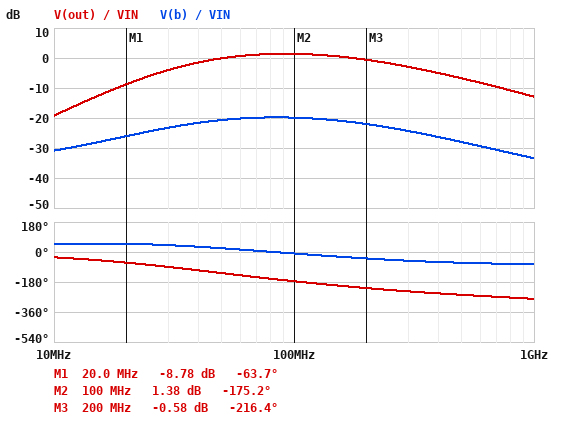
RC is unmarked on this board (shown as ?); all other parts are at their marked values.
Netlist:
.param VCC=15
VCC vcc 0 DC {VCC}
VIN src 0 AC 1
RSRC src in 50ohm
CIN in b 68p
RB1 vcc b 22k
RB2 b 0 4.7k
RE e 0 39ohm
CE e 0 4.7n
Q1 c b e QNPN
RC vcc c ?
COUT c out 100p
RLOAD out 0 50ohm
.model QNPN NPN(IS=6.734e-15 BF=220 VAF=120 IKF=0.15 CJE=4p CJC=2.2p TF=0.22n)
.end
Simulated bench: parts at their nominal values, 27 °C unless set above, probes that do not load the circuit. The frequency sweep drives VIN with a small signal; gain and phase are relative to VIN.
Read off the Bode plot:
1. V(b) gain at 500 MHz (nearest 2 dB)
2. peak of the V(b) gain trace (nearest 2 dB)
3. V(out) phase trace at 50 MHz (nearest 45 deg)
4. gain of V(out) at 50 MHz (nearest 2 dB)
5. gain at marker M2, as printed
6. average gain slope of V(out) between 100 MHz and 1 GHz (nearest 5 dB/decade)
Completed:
-28 dB
-20 dB
-135 deg
0 dB
1.38 dB
-15 dB/decade
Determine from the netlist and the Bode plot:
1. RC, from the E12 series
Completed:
1 kΩ
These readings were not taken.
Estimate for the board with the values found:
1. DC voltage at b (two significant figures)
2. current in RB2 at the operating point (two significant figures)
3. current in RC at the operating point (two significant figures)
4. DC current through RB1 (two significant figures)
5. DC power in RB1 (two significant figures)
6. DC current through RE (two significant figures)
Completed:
1.3 V
280 µA
14 mA
620 µA
8.5 mW
15 mA
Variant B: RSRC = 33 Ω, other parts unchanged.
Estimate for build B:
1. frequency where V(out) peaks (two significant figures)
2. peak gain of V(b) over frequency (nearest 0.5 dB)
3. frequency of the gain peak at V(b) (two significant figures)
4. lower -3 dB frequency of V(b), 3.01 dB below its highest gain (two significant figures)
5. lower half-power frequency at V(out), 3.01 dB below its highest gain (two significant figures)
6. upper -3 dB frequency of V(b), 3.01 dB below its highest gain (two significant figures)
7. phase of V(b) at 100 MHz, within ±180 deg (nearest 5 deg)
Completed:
110 MHz
-17.5 dB
100 MHz
39 MHz
46 MHz
270 MHz
0 deg
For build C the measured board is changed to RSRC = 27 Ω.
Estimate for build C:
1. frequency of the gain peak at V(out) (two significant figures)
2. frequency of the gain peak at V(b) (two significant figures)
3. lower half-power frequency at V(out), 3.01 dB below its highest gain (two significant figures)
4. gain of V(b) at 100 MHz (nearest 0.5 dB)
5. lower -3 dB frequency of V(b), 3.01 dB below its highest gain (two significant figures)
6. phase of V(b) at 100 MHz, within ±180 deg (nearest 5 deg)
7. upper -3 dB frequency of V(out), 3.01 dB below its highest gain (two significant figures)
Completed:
120 MHz
110 MHz
49 MHz
-16.5 dB
43 MHz
5 deg
300 MHz
